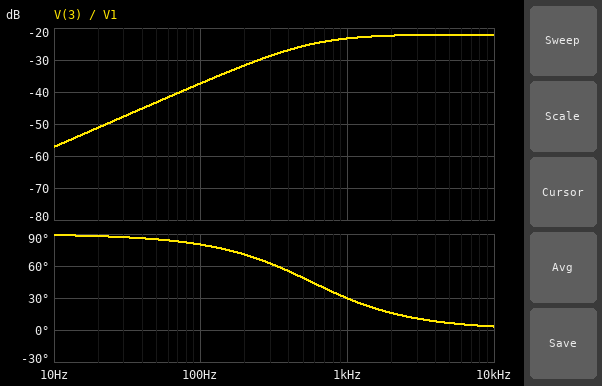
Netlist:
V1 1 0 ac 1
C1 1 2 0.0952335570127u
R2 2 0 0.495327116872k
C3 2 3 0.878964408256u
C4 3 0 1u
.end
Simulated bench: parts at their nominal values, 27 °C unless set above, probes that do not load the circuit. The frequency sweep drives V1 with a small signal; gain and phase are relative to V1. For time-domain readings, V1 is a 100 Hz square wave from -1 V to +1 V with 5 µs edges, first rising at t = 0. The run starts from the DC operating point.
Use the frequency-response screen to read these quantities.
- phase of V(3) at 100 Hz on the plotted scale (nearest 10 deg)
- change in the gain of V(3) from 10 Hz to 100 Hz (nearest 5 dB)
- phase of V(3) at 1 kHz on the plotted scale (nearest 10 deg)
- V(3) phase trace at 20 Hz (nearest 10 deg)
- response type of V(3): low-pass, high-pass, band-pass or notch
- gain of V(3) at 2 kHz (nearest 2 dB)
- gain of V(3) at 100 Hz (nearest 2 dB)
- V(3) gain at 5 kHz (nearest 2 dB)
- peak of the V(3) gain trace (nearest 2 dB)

80 deg
20 dB
30 deg
90 deg
high-pass
-22 dB
-38 dB
-22 dB
-22 dB
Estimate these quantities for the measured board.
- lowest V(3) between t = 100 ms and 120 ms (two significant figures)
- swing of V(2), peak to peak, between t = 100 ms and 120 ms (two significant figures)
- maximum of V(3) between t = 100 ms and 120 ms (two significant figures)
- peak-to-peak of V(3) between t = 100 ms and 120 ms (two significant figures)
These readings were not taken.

-160 mV
670 mV
160 mV
310 mV
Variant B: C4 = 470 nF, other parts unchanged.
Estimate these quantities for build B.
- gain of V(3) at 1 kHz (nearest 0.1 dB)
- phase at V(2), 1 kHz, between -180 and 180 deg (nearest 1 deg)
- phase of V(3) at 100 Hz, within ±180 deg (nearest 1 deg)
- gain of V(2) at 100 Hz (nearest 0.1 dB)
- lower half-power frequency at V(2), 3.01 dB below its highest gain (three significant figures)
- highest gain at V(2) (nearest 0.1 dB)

-18.4 dB
39 deg
83 deg
-30.6 dB
800 Hz
-12.5 dB
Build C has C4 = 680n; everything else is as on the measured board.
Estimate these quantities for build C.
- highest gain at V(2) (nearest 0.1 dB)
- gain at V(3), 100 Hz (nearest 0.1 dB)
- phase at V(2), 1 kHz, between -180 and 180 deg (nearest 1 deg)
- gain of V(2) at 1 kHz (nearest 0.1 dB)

-14.0 dB
-35.6 dB
34 deg
-15.6 dB
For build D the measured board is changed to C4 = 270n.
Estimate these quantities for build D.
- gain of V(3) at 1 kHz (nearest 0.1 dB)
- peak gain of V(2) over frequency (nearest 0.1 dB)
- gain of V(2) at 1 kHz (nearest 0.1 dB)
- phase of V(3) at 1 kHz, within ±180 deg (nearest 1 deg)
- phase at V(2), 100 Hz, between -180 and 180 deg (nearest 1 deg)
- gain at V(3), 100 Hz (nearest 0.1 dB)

-15.6 dB
-10.0 dB
-13.3 dB
47 deg
85 deg
-32.9 dB
